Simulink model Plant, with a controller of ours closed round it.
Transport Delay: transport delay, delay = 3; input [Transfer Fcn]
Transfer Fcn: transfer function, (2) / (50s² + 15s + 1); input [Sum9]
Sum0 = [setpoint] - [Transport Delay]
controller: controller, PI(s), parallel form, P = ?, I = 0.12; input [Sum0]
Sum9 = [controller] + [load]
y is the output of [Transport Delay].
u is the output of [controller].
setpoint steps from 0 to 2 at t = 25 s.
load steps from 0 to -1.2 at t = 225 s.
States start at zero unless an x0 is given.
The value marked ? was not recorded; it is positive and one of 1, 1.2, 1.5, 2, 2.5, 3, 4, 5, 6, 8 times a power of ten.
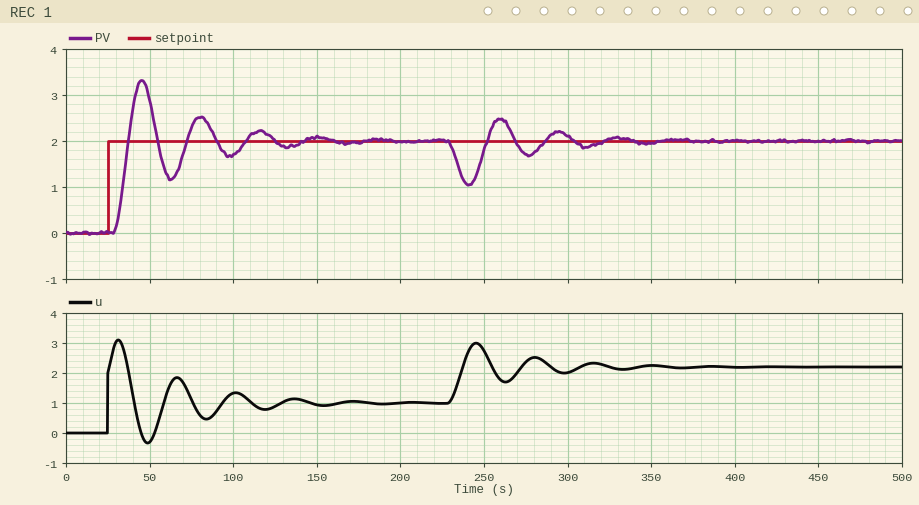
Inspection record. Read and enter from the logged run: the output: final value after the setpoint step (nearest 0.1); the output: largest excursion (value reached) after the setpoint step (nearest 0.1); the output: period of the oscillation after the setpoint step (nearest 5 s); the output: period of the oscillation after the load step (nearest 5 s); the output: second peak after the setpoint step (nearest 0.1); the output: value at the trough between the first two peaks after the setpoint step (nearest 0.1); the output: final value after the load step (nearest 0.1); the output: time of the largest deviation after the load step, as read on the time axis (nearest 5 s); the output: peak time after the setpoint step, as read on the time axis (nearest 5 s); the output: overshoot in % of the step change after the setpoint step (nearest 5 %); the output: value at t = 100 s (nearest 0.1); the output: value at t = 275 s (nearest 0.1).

2.0
3.3
35 s
35 s
2.5
1.2
2.0
240 s
45 s
65 %
1.7
1.7
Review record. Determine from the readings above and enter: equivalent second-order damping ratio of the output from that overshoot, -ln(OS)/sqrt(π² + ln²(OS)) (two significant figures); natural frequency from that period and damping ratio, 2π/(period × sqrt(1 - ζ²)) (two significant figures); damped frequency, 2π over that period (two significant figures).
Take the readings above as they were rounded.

0.14
0.18 rad/s
0.18 rad/s
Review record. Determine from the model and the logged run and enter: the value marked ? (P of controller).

1
